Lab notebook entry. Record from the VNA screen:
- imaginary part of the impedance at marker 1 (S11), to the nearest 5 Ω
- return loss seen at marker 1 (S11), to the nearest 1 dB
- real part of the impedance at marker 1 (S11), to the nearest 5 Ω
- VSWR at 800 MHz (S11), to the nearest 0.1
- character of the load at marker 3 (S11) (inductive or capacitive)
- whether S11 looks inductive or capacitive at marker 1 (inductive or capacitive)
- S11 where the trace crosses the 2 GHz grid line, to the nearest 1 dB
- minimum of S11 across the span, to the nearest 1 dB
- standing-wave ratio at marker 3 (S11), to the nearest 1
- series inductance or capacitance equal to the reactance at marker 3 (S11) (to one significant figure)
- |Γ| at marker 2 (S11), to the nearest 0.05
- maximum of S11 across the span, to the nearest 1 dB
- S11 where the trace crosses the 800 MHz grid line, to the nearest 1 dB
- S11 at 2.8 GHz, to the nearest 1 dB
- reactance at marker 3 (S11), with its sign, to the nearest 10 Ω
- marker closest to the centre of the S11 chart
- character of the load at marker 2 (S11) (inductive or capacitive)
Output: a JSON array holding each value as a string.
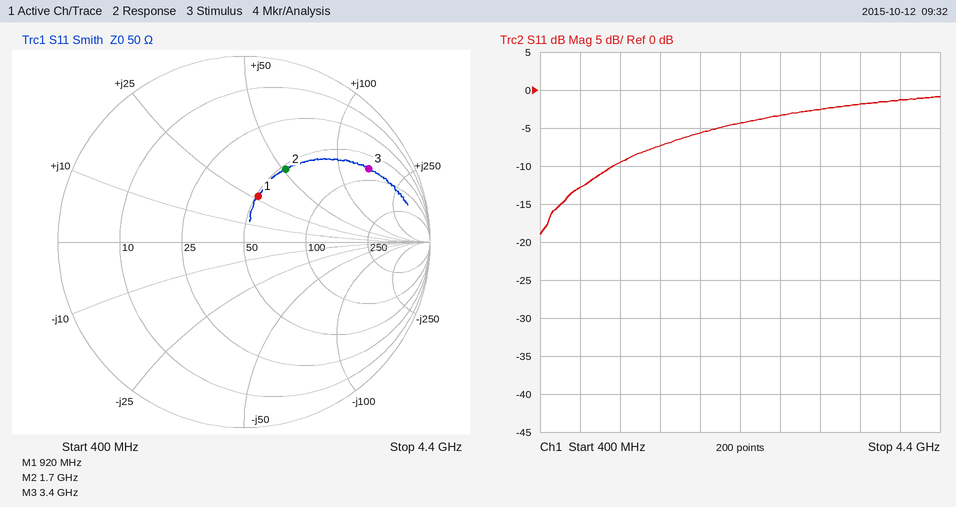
["+25 Ω", "12 dB", "50 Ω", "1.6", "inductive", "inductive", "-6 dB", "-19 dB", "8", "7 nH", "0.45", "-1 dB", "-13 dB", "-3 dB", "+150 Ω", "marker 1", "inductive"]
